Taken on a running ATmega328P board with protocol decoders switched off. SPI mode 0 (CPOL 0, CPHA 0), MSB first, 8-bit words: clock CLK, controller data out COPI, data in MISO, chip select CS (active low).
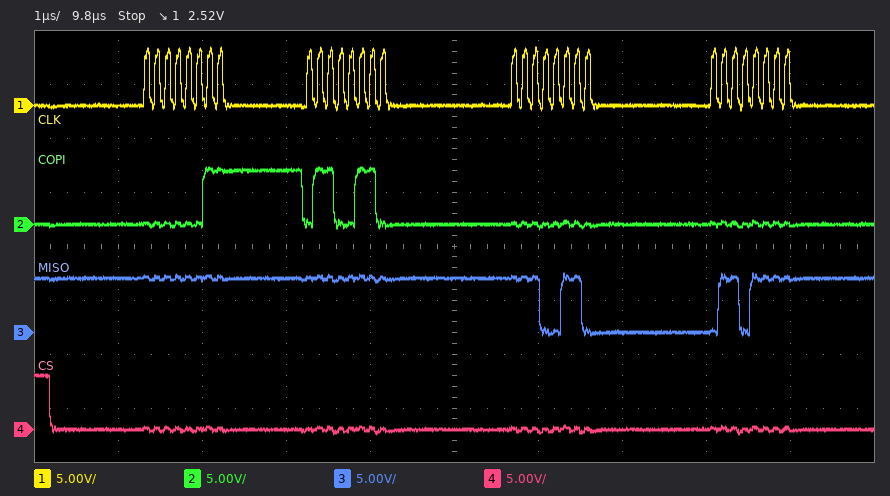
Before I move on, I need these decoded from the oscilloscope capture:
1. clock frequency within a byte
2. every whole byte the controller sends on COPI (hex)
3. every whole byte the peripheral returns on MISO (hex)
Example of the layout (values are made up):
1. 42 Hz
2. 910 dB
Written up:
1. 8 MHz
2. 0x03 0x66 0x00 0x00
3. 0xFF 0xFF 0xE6 0x6F
